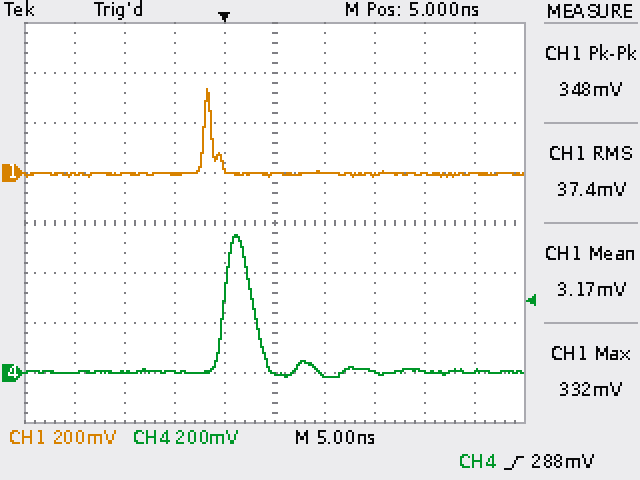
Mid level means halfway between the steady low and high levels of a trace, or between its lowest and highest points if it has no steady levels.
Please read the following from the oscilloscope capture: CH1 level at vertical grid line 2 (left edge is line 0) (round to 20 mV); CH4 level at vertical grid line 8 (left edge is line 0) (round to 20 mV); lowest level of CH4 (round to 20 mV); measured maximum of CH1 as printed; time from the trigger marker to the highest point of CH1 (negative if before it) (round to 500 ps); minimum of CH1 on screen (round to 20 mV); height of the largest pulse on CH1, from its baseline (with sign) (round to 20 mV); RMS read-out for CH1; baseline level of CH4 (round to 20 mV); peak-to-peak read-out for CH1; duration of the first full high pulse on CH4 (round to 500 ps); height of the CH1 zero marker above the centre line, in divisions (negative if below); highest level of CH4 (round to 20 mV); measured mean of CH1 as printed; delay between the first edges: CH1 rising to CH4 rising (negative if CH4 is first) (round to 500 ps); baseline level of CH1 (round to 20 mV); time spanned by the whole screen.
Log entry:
0 mV
0 mV
-20 mV
332 mV
-1.5 ns
-20 mV
+340 mV
37.4 mV
0 mV
348 mV
3.0 ns
+1.0 div
560 mV
3.17 mV
+2.0 ns
0 mV
50 ns
